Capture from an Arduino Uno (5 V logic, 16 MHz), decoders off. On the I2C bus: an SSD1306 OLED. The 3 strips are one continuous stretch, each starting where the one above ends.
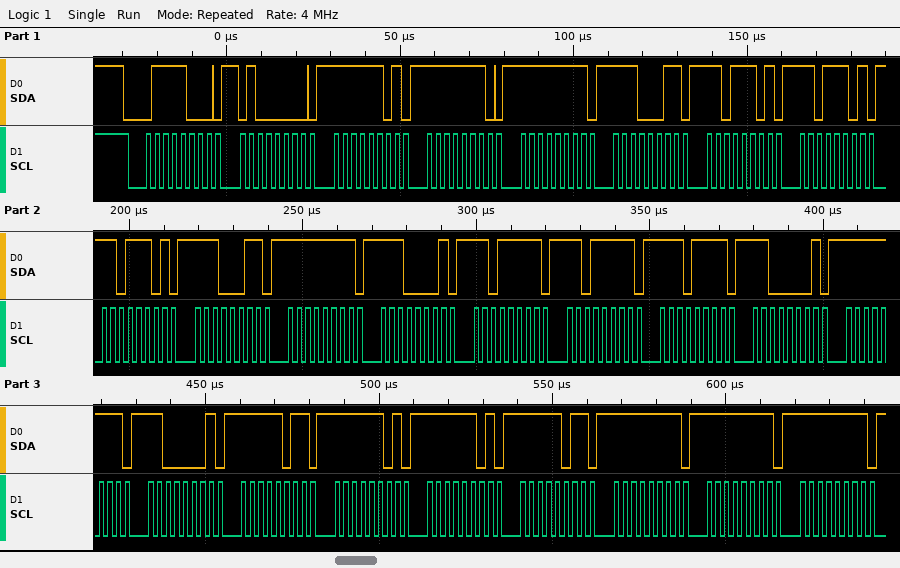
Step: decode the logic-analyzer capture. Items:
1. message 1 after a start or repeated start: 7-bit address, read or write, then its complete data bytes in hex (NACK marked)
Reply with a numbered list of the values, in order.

1. 0x3C write: 40 FD FE FF E3 DD DD DD E3 FF E1 DF DF EF C1 FF C1 FB FD FD FB FF FF FF
